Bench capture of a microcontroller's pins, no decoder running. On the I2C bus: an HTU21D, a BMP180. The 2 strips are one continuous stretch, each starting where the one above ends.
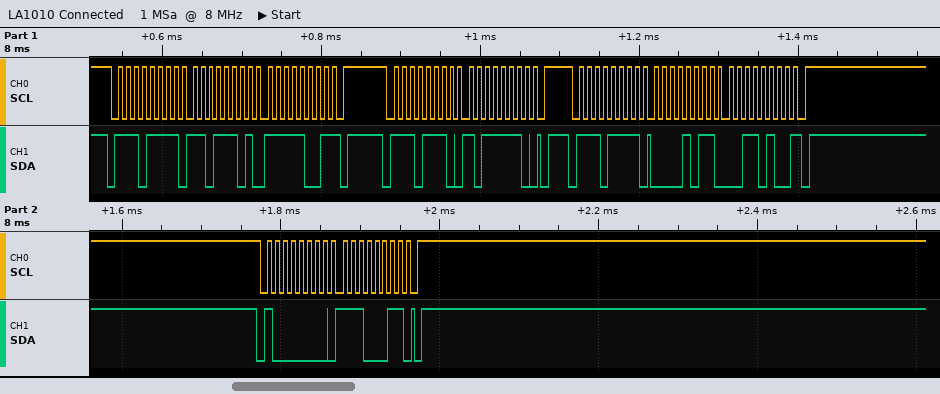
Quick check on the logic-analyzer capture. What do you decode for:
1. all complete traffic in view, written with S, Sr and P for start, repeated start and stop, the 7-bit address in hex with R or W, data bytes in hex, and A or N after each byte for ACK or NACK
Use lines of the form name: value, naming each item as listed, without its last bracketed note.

all complete traffic in view, written with S, Sr and P for start, repeated start and stop, the 7-bit address in hex with R or W, data bytes in hex, and A or N after each byte for ACK or NACK: S 77R A DD A F9 N P S 77W A BE A P S 77R A 0B A 34 N P S 40W A E3 A P
